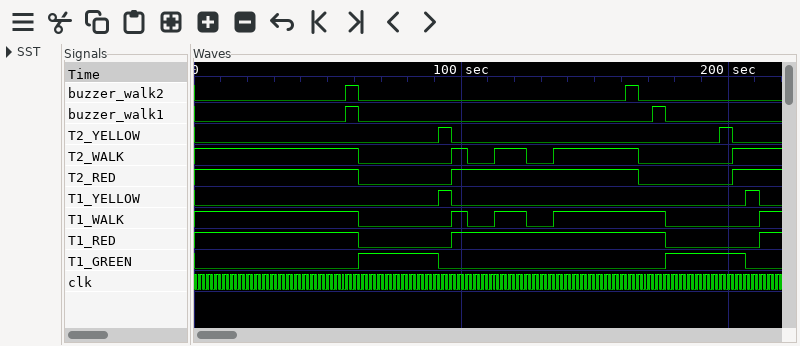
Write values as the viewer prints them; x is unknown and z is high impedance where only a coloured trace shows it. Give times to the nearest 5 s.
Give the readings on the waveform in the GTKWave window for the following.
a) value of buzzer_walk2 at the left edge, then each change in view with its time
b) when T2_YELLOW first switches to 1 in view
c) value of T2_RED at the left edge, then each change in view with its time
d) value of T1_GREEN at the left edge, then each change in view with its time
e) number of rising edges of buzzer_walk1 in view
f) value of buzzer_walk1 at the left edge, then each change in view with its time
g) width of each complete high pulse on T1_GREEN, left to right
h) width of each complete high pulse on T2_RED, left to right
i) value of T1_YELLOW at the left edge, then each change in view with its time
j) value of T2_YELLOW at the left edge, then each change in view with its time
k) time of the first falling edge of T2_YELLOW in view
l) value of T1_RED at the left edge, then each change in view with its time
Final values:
0, 1 at 55 s, 0 at 60 s, 1 at 160 s, 0 at 165 s
90 s
1, 0 at 60 s, 1 at 95 s, 0 at 165 s, 1 at 200 s
0, 1 at 60 s, 0 at 90 s, 1 at 175 s, 0 at 205 s
2
0, 1 at 55 s, 0 at 60 s, 1 at 170 s, 0 at 175 s
30 s, 30 s
70 s
0, 1 at 90 s, 0 at 95 s, 1 at 205 s, 0 at 210 s
0, 1 at 90 s, 0 at 95 s, 1 at 195 s, 0 at 200 s
95 s
1, 0 at 60 s, 1 at 95 s, 0 at 175 s, 1 at 210 s
